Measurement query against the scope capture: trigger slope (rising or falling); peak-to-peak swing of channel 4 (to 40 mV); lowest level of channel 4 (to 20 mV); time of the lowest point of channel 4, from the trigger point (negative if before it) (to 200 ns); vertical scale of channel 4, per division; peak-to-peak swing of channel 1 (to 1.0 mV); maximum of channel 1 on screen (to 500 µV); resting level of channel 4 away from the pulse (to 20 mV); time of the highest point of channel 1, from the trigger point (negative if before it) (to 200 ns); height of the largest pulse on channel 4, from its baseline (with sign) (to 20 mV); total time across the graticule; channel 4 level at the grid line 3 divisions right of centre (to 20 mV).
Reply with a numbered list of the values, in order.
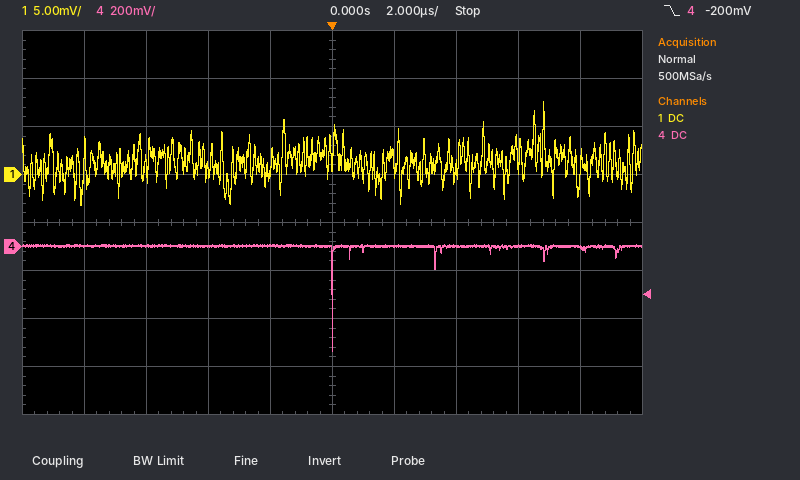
1. falling
2. 440 mV
3. -440 mV
4. 0.0 µs
5. 200 mV
6. 11.0 mV
7. 7.5 mV
8. 0 mV
9. +6.8 µs
10. -440 mV
11. 20 µs
12. 0 mV
